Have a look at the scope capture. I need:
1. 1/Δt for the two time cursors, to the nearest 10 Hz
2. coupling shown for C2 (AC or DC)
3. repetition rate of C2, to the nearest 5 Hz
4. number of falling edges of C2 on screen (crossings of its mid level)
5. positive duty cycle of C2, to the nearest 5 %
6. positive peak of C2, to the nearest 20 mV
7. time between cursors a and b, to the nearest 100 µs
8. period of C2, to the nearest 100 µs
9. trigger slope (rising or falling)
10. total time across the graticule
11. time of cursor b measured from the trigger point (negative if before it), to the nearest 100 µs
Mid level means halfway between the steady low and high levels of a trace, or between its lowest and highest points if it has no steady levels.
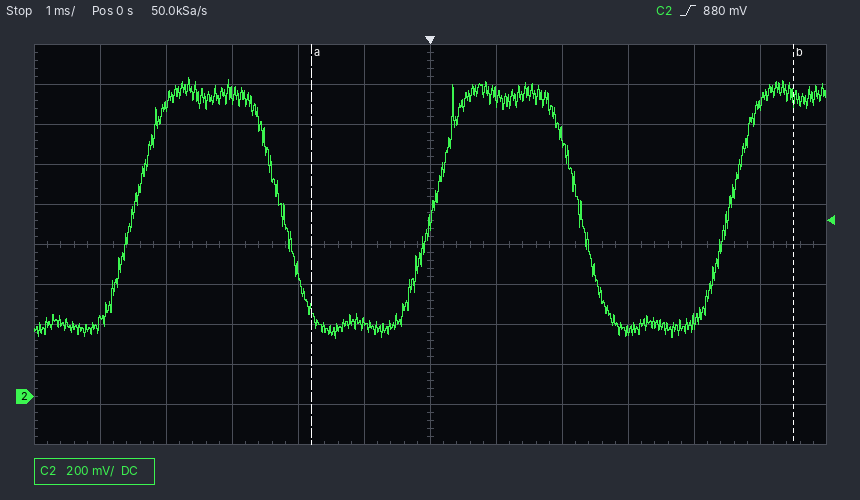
140 Hz
DC
220 Hz
2
50 %
1.60 V
7.3 ms
4.5 ms
rising
12 ms
+5.5 ms
